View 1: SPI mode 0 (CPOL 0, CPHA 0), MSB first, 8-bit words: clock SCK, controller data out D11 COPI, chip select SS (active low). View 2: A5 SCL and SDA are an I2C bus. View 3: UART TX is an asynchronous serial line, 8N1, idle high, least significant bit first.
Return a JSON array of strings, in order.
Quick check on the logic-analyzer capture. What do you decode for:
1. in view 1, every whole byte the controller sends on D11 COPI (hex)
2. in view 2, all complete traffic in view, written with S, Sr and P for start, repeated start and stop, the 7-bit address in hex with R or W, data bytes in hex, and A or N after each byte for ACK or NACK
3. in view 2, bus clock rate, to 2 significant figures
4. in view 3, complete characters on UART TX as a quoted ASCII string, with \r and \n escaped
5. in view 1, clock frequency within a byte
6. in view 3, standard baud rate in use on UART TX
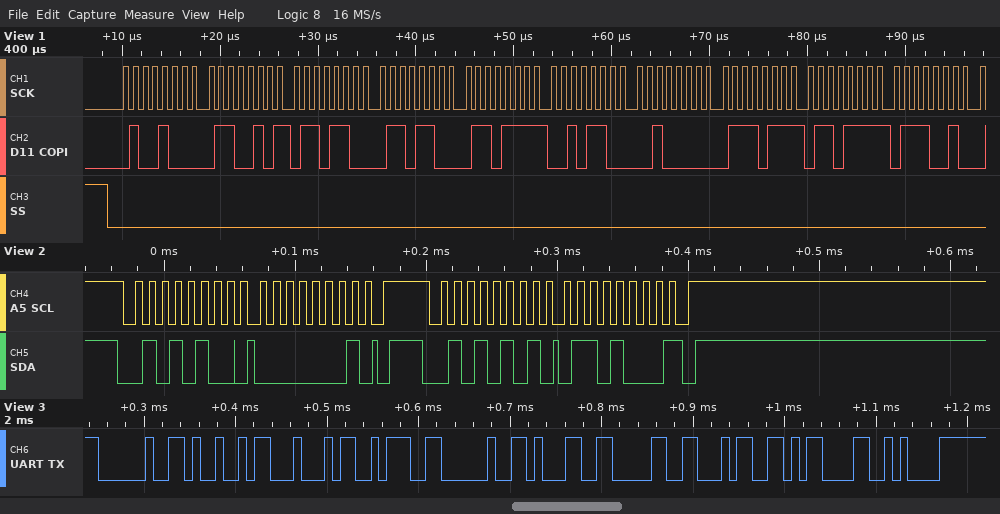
["48 65 6C 6C 6F 2C 20 77 6F 72", "S 2AW A 01 A P S 2AR A 68 N P", "100 kHz", "\" ID: 104\\r\\n\"", "1 MHz", "115200 baud"]
